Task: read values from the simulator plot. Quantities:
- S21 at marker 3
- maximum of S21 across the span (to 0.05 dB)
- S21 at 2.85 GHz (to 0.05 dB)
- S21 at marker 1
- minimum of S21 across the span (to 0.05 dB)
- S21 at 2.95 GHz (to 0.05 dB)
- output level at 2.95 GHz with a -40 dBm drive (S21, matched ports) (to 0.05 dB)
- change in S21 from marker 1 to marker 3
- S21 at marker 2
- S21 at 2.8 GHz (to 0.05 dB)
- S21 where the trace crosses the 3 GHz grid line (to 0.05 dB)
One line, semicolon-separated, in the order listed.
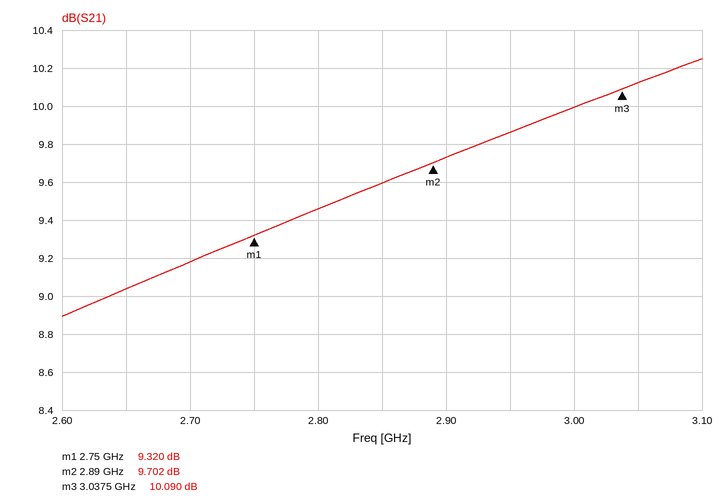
10.090 dB; 10.25 dB; 9.60 dB; 9.320 dB; 8.90 dB; 9.85 dB; -30.15 dBm; 0.770 dB; 9.702 dB; 9.45 dB; 10.00 dB
